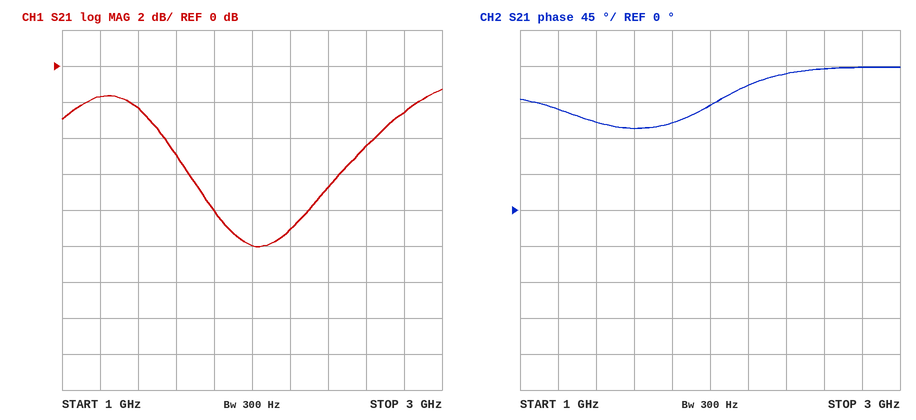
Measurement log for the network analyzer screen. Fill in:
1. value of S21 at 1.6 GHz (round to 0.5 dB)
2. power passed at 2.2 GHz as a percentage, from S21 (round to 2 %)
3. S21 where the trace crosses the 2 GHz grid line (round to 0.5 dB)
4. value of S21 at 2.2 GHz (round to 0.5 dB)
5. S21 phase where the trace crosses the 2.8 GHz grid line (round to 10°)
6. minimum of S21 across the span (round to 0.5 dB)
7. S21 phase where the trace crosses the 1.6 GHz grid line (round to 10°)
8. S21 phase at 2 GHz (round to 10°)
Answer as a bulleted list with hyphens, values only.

- -5.0 dB
- 12 %
- -10.0 dB
- -9.0 dB
- 180°
- -10.0 dB
- 100°
- 130°
